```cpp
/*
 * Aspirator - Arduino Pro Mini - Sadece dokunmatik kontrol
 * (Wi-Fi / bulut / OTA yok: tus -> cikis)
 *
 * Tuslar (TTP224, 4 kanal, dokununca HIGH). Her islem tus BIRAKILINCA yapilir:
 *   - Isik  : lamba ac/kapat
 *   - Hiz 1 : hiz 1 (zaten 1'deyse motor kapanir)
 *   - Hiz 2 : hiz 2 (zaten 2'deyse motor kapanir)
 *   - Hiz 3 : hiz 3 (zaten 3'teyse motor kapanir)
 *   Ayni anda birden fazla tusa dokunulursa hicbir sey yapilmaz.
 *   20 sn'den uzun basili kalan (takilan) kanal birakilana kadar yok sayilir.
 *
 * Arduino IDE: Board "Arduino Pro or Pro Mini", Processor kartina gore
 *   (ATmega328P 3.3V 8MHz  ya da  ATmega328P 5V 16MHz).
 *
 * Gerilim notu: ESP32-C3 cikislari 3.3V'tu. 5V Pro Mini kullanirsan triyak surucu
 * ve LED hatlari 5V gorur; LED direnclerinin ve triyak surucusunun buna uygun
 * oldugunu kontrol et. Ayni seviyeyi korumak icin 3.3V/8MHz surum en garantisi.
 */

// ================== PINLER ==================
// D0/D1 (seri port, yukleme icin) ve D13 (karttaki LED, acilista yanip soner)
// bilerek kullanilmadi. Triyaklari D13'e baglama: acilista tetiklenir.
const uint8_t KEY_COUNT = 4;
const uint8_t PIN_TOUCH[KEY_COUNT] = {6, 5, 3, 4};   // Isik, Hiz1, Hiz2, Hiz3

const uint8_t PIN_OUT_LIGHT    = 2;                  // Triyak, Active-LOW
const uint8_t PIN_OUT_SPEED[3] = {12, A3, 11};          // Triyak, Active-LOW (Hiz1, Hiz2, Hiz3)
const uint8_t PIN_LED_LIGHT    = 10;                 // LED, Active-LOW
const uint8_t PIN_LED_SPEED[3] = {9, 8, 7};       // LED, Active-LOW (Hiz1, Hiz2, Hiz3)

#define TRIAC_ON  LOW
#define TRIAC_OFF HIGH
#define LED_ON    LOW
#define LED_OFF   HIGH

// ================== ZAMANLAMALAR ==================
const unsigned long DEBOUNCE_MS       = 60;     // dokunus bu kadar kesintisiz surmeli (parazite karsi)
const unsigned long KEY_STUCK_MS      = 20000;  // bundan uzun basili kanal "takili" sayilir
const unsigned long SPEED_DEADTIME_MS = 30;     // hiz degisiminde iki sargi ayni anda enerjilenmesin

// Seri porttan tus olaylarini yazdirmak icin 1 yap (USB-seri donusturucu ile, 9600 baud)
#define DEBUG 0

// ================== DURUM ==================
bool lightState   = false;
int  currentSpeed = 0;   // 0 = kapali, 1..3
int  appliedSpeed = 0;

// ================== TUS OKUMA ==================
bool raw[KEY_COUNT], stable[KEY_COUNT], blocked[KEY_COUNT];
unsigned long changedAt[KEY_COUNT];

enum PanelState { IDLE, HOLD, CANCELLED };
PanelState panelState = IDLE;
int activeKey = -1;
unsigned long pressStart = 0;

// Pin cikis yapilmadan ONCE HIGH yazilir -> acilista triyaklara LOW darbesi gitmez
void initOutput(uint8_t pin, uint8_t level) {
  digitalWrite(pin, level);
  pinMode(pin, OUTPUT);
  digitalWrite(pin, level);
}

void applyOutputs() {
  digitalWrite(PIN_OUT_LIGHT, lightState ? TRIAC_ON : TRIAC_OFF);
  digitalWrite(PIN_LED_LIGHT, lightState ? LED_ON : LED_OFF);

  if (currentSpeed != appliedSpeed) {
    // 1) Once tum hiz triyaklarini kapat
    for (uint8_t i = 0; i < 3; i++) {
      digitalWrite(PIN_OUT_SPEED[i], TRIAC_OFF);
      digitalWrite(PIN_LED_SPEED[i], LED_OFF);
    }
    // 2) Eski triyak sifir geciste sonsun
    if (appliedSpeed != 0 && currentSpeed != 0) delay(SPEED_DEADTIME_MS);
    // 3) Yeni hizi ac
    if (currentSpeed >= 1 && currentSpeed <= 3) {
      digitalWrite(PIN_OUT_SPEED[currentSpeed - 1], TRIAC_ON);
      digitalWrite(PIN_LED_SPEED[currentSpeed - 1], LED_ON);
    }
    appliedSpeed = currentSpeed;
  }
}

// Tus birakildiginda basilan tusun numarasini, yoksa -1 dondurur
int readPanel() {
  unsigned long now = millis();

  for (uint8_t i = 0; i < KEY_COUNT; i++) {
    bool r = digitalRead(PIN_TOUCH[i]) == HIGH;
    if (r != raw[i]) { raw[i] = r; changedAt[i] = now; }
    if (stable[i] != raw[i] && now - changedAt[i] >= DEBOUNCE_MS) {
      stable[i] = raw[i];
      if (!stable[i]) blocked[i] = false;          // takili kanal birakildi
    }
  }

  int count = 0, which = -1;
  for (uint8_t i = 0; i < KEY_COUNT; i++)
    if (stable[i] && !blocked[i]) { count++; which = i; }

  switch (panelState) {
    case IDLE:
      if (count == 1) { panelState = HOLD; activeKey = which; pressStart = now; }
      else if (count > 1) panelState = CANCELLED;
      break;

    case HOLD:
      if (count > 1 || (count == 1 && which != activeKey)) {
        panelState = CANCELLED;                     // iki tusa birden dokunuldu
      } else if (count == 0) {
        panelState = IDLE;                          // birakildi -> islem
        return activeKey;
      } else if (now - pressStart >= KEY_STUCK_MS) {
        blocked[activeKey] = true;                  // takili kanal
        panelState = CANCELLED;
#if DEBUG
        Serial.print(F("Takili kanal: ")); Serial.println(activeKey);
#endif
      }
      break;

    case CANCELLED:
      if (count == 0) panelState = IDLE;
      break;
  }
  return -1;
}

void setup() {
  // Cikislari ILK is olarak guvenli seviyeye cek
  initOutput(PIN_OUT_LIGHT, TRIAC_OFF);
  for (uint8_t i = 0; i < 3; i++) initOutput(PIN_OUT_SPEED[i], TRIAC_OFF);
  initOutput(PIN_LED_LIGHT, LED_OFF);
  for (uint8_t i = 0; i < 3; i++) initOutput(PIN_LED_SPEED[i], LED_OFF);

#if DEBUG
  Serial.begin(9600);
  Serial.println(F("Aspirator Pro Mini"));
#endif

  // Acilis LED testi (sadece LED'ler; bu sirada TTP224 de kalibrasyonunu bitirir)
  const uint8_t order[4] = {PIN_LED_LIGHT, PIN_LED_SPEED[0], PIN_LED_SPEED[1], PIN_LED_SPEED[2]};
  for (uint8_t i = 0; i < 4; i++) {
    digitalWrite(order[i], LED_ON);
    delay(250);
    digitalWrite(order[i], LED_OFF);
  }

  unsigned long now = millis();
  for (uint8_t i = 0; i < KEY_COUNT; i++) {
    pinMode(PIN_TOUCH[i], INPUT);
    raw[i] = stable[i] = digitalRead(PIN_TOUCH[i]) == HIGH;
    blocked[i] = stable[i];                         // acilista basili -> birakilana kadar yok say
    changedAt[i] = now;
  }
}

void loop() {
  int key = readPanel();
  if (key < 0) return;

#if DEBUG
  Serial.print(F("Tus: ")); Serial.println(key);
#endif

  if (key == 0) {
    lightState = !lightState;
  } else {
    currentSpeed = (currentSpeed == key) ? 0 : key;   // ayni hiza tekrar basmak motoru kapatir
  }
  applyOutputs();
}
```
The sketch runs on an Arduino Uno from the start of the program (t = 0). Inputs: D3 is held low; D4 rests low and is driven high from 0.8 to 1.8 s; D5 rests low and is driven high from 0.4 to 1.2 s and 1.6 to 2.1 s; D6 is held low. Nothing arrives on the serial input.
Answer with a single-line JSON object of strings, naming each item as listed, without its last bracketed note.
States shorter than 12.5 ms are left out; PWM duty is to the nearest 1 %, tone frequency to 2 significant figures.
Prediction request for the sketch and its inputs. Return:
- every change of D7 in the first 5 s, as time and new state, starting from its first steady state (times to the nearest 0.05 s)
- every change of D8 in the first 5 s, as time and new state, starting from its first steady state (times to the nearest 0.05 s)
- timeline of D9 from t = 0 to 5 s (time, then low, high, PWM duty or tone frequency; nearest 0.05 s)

{"every change of D7 in the first 5 s, as time and new state, starting from its first steady state": "0 s high; 0.75 s low; 1 s high", "every change of D8 in the first 5 s, as time and new state, starting from its first steady state": "0 s high; 0.5 s low; 0.75 s high", "timeline of D9 from t = 0 to 5 s": "0 s high; 0.25 s low; 0.5 s high; 2.15 s low"}
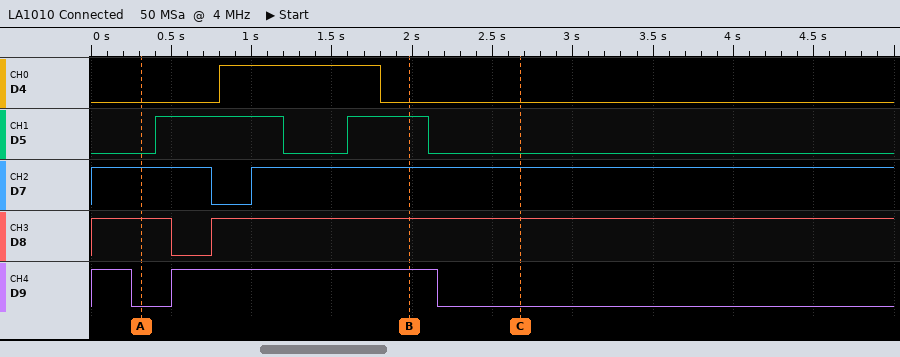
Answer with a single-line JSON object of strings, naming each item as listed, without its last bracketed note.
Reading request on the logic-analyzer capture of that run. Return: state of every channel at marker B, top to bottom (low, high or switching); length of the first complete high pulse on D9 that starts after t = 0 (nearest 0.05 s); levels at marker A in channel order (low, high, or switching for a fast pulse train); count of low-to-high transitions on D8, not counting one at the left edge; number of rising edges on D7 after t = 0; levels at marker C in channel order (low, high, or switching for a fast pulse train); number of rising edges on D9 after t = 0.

{"state of every channel at marker B, top to bottom": "D4 low, D5 high, D7 high, D8 high, D9 high", "length of the first complete high pulse on D9 that starts after t = 0": "1.65 s", "levels at marker A in channel order": "D4 low, D5 low, D7 high, D8 high, D9 low", "count of low-to-high transitions on D8, not counting one at the left edge": "1", "number of rising edges on D7 after t = 0": "1", "levels at marker C in channel order": "D4 low, D5 low, D7 high, D8 high, D9 low", "number of rising edges on D9 after t = 0": "1"}
